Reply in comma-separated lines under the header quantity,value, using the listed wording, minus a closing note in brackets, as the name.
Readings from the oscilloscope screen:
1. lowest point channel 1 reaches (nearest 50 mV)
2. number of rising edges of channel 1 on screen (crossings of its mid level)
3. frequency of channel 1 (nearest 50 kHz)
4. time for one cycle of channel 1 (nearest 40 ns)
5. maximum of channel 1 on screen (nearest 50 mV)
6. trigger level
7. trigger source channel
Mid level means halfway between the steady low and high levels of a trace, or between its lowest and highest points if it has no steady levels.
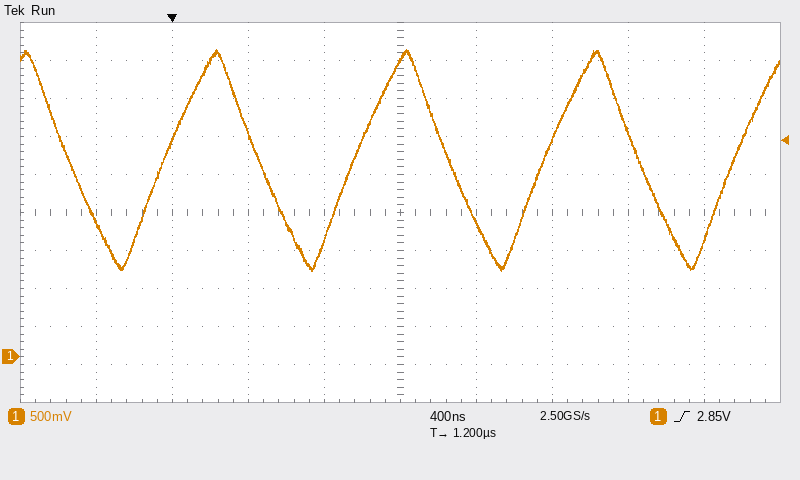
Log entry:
quantity,value
lowest point channel 1 reaches,1.10 V
number of rising edges of channel 1 on screen,4
frequency of channel 1,1.00 MHz
time for one cycle of channel 1,1.00 µs
maximum of channel 1 on screen,4.05 V
trigger level,2.85 V
trigger source channel,channel 1
